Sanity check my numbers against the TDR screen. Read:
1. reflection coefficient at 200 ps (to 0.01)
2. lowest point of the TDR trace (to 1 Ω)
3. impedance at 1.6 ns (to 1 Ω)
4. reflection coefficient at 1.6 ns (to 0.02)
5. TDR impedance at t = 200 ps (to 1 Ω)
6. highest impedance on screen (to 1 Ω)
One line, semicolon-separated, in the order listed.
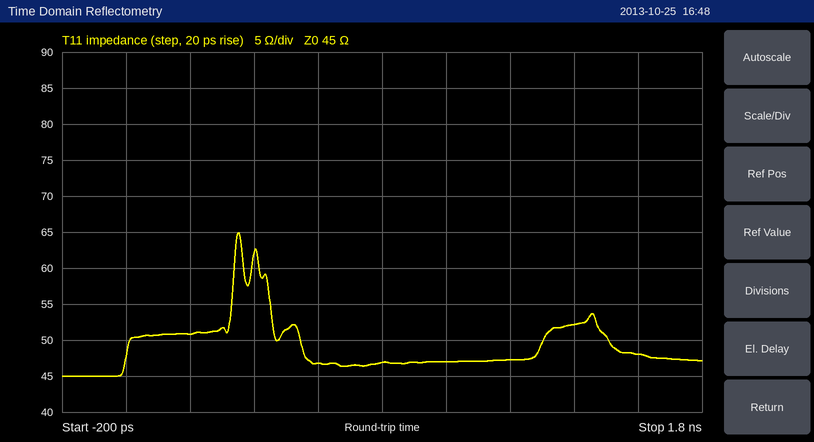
+0.06; 45 Ω; 48 Ω; +0.04; 51 Ω; 65 Ω
